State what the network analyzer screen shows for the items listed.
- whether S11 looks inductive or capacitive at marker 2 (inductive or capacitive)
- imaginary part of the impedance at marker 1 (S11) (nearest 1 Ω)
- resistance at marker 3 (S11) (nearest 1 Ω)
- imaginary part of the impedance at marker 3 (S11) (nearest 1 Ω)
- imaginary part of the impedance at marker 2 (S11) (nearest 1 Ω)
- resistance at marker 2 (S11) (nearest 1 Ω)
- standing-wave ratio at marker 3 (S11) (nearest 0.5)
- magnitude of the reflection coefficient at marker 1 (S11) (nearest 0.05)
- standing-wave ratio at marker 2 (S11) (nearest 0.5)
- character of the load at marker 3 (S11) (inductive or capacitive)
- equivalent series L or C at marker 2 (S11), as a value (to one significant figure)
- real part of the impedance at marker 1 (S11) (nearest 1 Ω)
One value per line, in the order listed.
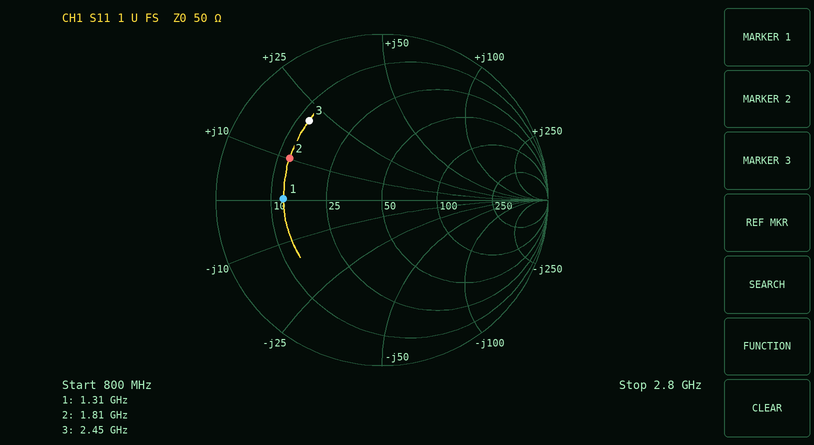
inductive
0 Ω
13 Ω
+21 Ω
+10 Ω
13 Ω
4.5
0.60
4.0
inductive
900 pH
13 Ω
